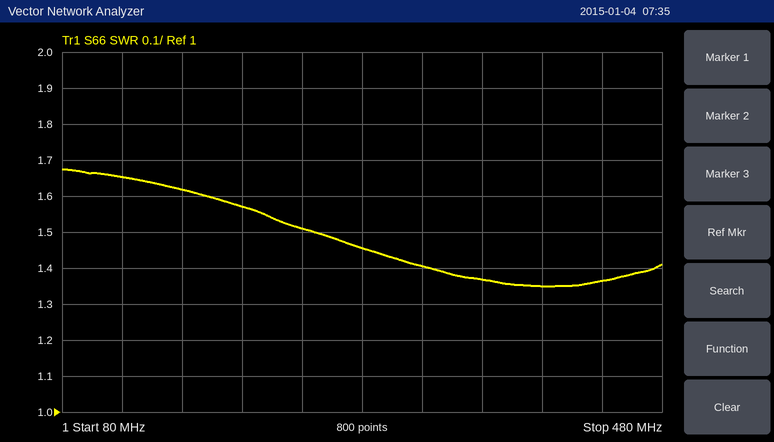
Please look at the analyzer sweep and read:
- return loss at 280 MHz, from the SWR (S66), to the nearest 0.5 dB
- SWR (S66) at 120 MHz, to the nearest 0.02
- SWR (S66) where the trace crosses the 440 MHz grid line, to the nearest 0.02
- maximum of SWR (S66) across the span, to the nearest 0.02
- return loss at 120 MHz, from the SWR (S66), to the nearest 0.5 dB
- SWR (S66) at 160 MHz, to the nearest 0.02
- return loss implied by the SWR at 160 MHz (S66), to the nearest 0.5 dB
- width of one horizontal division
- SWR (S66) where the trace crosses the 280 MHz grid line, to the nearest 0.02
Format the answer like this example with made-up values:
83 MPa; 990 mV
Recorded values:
14.5 dB; 1.66; 1.36; 1.68; 12.0 dB; 1.62; 12.5 dB; 40 MHz; 1.46
